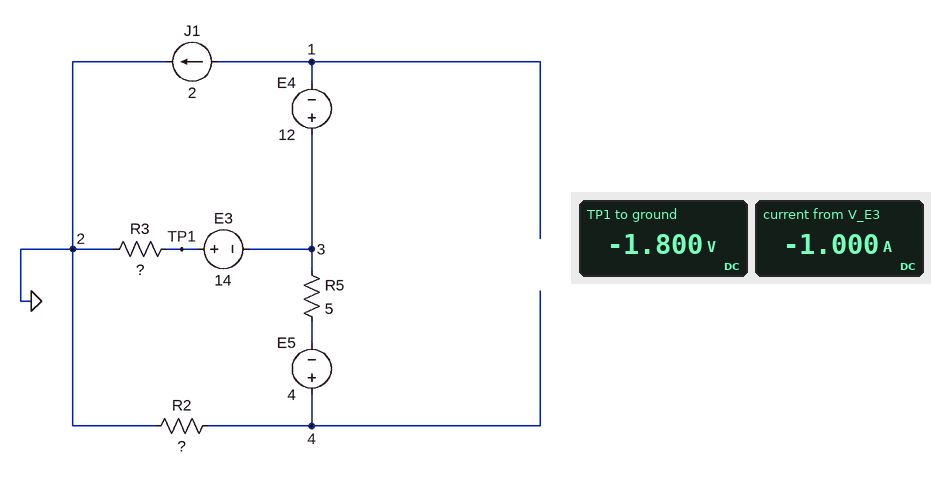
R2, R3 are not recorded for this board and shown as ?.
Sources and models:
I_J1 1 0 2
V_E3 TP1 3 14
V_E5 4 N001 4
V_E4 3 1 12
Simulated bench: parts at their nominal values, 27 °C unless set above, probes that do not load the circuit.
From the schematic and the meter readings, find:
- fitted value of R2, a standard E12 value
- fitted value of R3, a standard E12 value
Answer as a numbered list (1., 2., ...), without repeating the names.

1. 6.8 Ω
2. 1.8 Ω
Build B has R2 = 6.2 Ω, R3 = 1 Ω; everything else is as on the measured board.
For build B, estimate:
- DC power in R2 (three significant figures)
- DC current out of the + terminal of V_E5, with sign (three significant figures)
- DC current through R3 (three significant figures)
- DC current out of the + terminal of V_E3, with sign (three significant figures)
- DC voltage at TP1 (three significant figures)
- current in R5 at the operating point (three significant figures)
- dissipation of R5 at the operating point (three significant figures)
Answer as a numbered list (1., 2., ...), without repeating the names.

1. 6.00 W
2. -984 mA
3. 1.02 A
4. -1.02 A
5. -1.02 V
6. 984 mA
7. 4.84 W
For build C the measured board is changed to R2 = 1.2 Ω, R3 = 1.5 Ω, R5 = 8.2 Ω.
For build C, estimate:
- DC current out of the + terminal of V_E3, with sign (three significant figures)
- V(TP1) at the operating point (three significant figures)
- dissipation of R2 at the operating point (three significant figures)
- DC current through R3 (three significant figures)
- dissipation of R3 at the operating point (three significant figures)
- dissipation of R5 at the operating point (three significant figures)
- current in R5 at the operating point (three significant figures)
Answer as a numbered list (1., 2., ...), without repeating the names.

1. -807 mA
2. -1.21 V
3. 1.71 W
4. 807 mA
5. 978 mW
6. 11.7 W
7. 1.19 A
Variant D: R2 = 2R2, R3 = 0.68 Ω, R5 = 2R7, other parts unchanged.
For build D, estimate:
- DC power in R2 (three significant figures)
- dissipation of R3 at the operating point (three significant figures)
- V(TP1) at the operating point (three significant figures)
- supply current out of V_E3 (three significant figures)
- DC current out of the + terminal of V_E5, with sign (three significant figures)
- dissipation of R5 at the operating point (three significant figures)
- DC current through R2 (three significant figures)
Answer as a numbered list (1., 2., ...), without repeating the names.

1. 9.12 W
2. 874 µW
3. 24.4 mV
4. 35.8 mA
5. -2.04 A
6. 11.2 W
7. 2.04 A
